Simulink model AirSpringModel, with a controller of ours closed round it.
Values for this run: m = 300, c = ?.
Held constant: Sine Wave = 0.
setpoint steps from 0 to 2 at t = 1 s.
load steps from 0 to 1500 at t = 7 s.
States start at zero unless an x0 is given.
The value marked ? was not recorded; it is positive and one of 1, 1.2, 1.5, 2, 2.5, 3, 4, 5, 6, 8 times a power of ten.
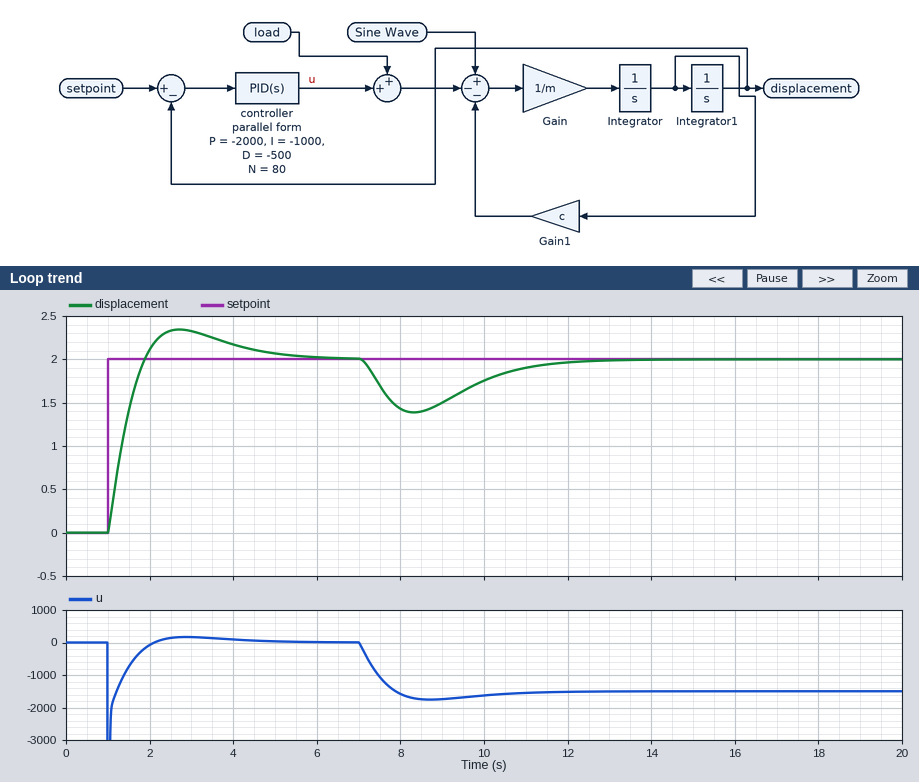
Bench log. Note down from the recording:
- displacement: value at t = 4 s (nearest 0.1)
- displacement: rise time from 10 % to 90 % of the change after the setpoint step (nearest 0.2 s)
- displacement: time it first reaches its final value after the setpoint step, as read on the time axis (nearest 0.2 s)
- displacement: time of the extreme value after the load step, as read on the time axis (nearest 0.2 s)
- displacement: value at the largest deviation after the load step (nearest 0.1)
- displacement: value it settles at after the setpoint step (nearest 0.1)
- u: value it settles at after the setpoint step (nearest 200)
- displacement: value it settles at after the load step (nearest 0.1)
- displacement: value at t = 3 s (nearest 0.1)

2.2
0.6 s
1.8 s
8.4 s
1.4
2.0
0
2.0
2.3
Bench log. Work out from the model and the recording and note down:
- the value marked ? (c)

800
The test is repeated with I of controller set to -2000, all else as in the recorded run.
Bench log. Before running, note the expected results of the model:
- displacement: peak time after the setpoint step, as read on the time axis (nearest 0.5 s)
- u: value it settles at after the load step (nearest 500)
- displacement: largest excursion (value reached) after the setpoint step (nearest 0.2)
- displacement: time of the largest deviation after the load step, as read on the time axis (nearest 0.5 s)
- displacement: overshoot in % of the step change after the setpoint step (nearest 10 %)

2.5 s
-1500
2.6
8.0 s
30 %
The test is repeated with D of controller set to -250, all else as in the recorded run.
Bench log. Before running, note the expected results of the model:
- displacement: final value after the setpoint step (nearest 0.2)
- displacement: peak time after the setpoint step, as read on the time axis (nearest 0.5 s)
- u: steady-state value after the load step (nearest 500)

2.0
2.5 s
-1500
